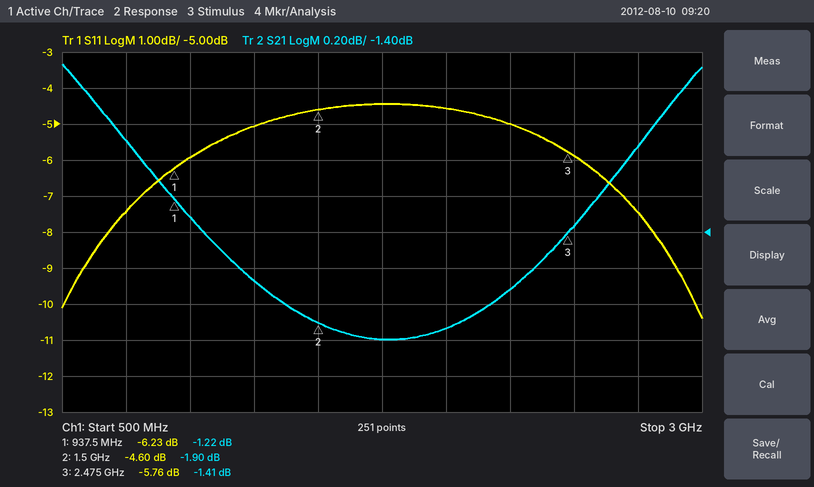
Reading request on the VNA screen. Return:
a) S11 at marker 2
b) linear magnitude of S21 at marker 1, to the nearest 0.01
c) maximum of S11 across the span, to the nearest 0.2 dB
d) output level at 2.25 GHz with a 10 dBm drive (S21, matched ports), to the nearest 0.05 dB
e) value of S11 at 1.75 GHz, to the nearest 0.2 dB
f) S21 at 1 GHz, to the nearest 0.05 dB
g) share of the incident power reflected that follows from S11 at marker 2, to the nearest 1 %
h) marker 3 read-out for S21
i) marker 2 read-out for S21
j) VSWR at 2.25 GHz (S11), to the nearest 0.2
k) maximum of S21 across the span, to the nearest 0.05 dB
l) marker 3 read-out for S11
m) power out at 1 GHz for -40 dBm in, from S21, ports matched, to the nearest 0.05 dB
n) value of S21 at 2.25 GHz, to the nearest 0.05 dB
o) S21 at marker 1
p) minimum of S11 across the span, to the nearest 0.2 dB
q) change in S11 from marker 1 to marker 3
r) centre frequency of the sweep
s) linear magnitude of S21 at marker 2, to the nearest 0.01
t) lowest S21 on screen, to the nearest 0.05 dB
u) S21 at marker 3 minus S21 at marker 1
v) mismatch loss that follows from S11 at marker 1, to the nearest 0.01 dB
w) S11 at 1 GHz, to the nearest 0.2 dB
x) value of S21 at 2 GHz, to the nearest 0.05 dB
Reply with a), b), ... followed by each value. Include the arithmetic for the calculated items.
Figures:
a) -4.60 dB
b) 10^(-1.22/20) ≈ 0.87
c) -4.4 dB
d) 10 dBm + (-1.70 dB) = 8.30 dBm
e) -4.4 dB
f) -1.30 dB
g) 10^(-4.6/10) ≈ 35 %
h) -1.41 dB
i) -1.90 dB
j) |Γ| = 10^(-5/20) = 0.5623; VSWR = (1 + 0.5623)/(1 − 0.5623) ≈ 3.6
k) -0.45 dB
l) -5.76 dB
m) -40 dBm + (-1.30 dB) = -41.30 dBm
n) -1.70 dB
o) -1.22 dB
p) -10.4 dB
q) -5.76 − (-6.23) = 0.47 dB
r) 1.75 GHz
s) 10^(-1.9/20) ≈ 0.80
t) -2.00 dB
u) -1.41 − (-1.22) = -0.19 dB
v) −10 log10(1 − 10^(-6.23/10)) ≈ 1.18 dB
w) -6.0 dB
x) -1.95 dB
